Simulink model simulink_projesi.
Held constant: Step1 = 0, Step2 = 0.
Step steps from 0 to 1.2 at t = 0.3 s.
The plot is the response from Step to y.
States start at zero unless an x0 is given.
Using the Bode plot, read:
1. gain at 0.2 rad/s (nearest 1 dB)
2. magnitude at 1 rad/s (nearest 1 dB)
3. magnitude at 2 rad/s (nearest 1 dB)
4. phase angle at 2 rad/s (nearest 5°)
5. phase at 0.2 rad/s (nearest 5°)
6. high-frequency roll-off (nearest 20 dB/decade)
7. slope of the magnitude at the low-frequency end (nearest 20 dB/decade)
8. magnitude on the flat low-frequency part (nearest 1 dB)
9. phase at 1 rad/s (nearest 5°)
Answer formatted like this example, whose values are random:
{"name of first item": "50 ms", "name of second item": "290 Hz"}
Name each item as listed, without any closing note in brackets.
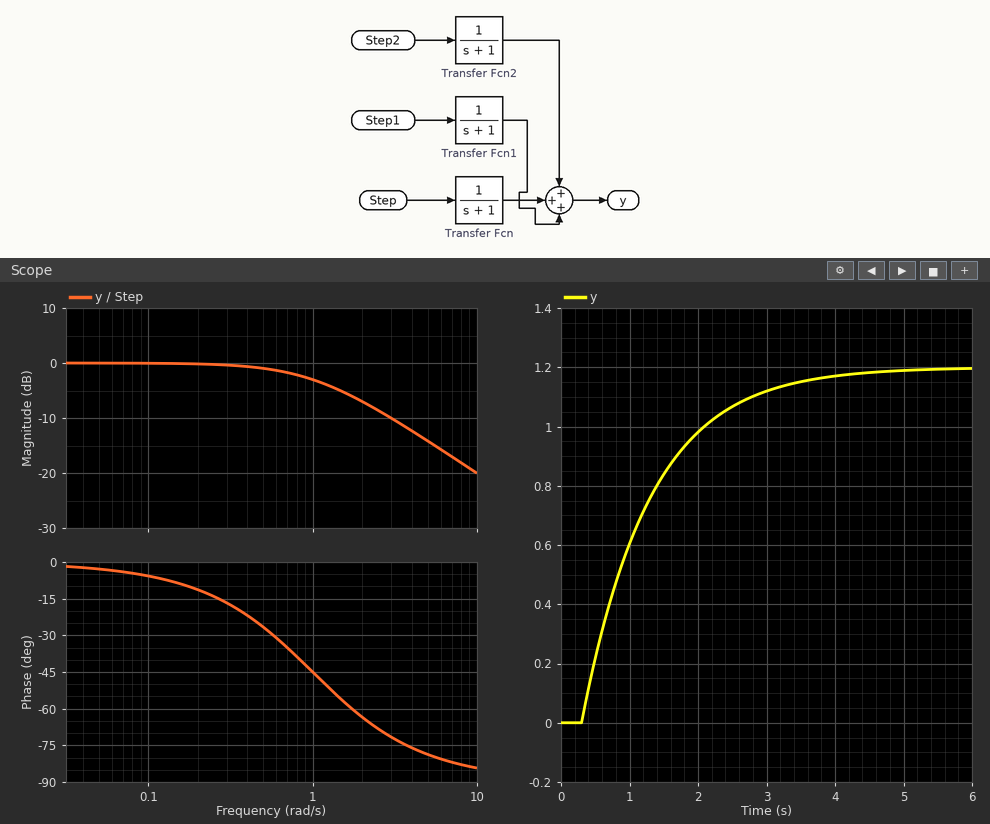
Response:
{"gain at 0.2 rad/s": "0 dB", "magnitude at 1 rad/s": "-3 dB", "magnitude at 2 rad/s": "-7 dB", "phase angle at 2 rad/s": "-65°", "phase at 0.2 rad/s": "-10°", "high-frequency roll-off": "-20 dB/decade", "slope of the magnitude at the low-frequency end": "0 dB/decade", "magnitude on the flat low-frequency part": "0 dB", "phase at 1 rad/s": "-45°"}
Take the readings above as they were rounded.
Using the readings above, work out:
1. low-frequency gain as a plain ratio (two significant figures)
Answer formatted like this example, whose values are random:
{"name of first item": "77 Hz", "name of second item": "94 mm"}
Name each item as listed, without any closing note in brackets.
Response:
{"low-frequency gain as a plain ratio": "1.0"}
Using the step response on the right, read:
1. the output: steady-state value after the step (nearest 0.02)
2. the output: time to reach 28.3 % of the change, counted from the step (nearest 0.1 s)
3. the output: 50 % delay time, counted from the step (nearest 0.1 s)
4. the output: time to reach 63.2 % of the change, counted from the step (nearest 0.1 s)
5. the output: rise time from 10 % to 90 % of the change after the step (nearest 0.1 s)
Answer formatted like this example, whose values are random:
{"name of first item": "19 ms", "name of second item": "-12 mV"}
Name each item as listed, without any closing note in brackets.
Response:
{"the output: steady-state value after the step": "1.20", "the output: time to reach 28.3 % of the change, counted from the step": "0.3 s", "the output: 50 % delay time, counted from the step": "0.7 s", "the output: time to reach 63.2 % of the change, counted from the step": "1.0 s", "the output: rise time from 10 % to 90 % of the change after the step": "2.2 s"}
